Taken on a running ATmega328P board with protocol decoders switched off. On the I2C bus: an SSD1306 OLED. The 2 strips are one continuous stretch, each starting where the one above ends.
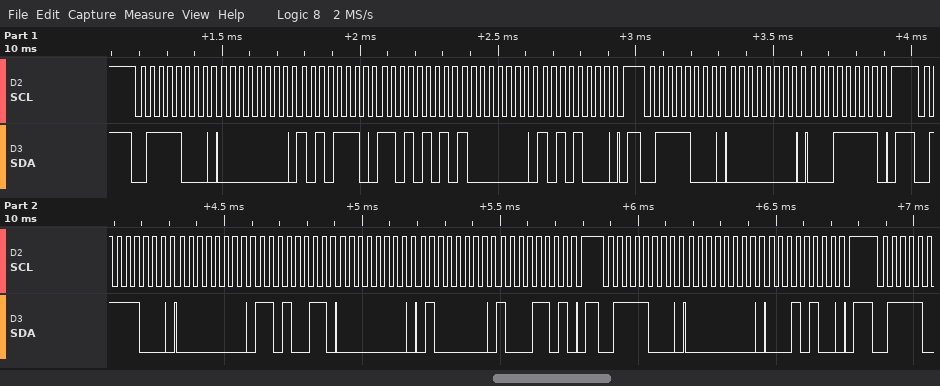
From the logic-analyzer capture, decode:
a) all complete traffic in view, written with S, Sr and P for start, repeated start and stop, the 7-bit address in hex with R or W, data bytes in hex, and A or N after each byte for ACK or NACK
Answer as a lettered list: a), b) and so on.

a) S 3CW A 00 A AE A D5 A 80 A A8 A P S 3CW A 00 A 1F A P S 3CW A 00 A D3 A 00 A 40 A 8D A P S 3CW A 00 A 14 A P
